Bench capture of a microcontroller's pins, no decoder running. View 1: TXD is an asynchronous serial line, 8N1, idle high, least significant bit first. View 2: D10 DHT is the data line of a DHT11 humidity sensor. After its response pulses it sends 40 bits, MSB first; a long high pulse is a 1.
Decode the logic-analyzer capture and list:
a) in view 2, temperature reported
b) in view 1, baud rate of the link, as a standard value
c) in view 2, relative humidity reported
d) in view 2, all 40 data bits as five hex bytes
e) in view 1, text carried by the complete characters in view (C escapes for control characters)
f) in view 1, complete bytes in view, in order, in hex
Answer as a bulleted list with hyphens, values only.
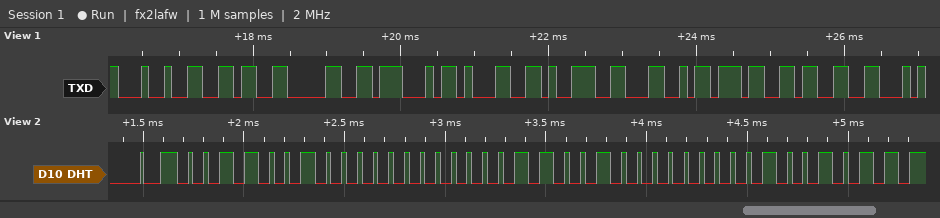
- 25.0 °C
- 9600 baud
- 50 %
- 32 00 19 00 4B
- "$60G19L73"
- 24 36 30 47 31 39 4C 37 33
